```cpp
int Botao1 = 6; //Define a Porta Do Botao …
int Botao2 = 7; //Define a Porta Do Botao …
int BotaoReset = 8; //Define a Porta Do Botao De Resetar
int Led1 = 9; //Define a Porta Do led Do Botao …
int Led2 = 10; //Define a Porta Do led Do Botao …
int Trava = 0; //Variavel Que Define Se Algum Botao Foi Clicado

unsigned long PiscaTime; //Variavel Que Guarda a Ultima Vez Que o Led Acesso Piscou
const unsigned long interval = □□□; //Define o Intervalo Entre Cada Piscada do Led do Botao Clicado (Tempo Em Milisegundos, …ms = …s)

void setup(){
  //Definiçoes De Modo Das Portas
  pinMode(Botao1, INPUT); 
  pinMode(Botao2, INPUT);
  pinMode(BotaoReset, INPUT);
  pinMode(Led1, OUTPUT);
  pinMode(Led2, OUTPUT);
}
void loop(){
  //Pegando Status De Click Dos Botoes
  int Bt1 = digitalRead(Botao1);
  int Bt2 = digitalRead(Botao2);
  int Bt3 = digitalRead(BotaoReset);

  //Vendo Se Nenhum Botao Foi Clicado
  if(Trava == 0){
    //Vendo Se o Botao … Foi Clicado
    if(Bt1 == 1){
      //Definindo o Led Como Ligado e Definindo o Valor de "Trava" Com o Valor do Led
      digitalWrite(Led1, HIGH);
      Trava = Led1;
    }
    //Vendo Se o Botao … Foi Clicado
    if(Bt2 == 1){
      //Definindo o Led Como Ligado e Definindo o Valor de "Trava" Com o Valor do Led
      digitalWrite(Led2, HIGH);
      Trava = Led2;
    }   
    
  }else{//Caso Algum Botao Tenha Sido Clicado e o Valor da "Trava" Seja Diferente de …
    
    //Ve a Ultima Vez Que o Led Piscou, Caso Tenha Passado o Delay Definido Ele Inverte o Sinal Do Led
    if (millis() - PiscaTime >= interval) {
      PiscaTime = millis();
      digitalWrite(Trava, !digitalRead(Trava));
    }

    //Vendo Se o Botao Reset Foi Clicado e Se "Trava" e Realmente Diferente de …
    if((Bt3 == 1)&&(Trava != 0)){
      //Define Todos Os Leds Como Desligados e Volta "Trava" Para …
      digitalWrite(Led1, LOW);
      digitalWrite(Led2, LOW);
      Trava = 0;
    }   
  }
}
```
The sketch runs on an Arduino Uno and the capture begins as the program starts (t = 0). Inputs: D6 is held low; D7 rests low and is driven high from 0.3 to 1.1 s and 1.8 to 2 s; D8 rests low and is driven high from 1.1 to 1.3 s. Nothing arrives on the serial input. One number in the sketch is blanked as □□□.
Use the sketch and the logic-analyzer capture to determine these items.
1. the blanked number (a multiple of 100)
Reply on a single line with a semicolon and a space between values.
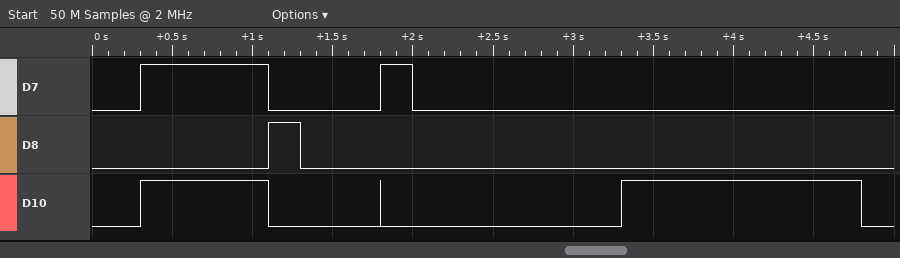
1500
